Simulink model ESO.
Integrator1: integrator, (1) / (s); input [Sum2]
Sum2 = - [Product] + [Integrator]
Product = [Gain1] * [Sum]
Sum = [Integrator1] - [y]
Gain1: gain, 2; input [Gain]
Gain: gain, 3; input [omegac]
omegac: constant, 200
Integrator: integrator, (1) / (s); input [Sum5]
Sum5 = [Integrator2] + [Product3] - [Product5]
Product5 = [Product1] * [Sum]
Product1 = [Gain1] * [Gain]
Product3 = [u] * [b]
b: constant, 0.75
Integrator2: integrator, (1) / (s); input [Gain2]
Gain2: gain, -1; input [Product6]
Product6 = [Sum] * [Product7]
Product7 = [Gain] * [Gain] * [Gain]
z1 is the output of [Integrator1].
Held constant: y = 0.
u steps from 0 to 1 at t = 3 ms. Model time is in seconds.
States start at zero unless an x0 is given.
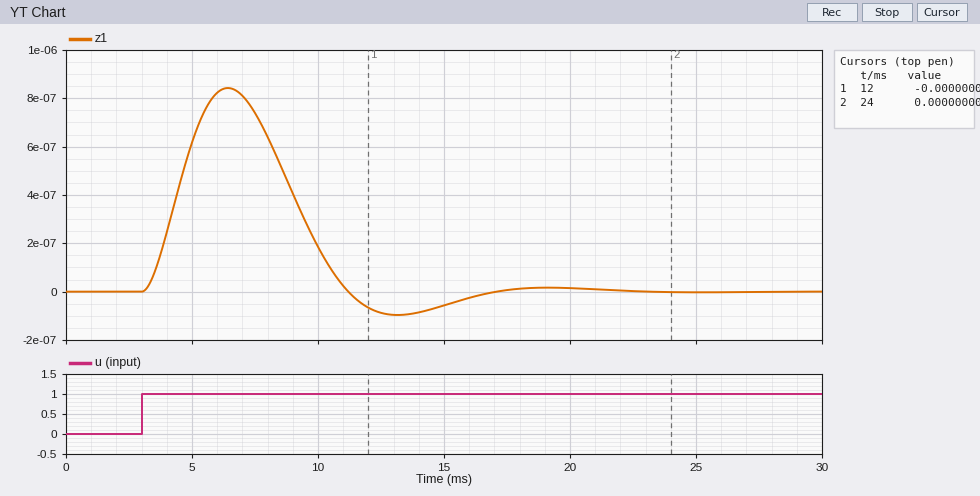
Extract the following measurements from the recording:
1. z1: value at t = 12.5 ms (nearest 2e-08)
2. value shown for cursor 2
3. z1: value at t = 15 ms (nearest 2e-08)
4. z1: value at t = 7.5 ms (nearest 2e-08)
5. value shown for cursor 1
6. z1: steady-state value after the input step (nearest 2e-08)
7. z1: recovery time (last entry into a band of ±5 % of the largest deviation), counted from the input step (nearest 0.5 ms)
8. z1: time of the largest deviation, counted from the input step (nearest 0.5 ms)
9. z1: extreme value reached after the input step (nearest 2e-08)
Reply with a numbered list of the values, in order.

1. -0.00000008
2. 0.000000000
3. -0.00000006
4. 0.00000074
5. -0.000000065
6. 0.00000000
7. 12.5 ms
8. 3.5 ms
9. 0.00000084
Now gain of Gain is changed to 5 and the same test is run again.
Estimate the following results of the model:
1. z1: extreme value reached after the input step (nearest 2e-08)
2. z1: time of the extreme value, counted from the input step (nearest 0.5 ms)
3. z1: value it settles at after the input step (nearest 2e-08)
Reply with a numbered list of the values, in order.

1. 0.00000030
2. 2.0 ms
3. 0.00000000
